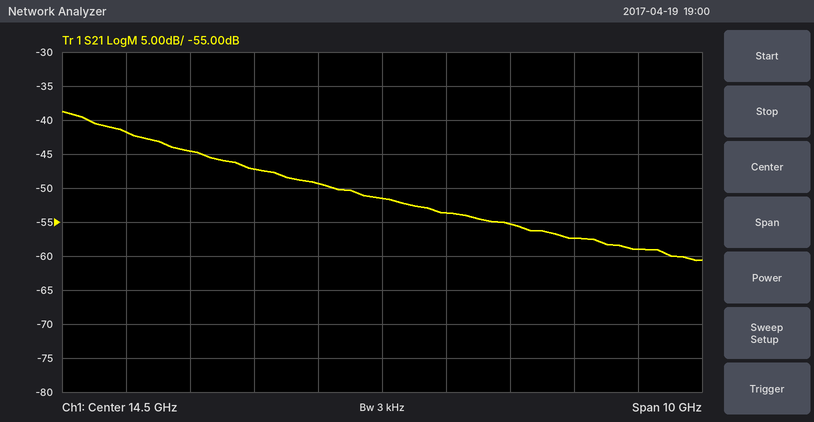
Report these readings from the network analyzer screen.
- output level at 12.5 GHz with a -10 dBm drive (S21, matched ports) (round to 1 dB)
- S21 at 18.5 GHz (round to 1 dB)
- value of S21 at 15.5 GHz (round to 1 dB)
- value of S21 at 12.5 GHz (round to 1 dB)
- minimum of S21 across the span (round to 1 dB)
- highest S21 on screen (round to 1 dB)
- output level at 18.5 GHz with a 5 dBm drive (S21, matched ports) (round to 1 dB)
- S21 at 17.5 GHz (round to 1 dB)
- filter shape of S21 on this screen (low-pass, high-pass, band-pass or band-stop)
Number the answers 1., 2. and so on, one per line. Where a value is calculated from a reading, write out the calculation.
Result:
1. -10 dBm + (-47 dB) = -57 dBm
2. -59 dB
3. -54 dB
4. -47 dB
5. -61 dB
6. -39 dB
7. 5 dBm + (-59 dB) = -54 dBm
8. -57 dB
9. low-pass
